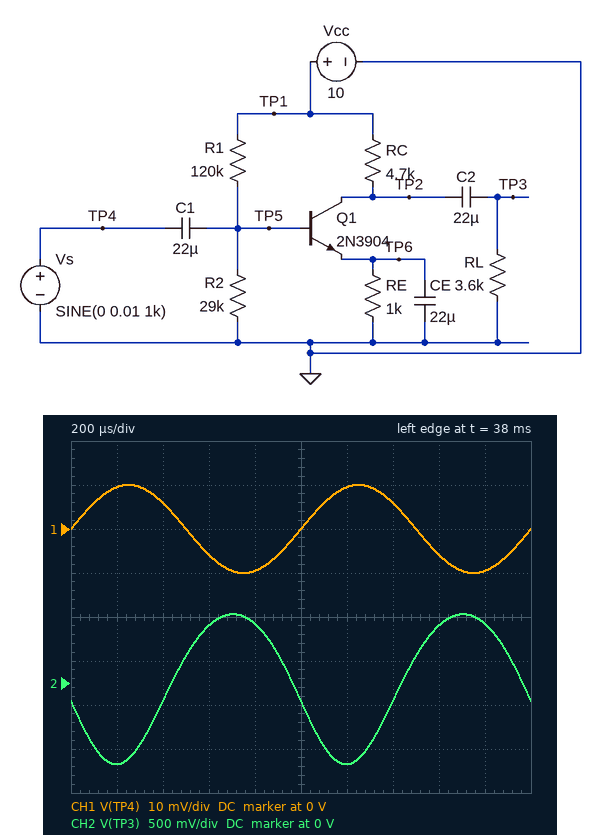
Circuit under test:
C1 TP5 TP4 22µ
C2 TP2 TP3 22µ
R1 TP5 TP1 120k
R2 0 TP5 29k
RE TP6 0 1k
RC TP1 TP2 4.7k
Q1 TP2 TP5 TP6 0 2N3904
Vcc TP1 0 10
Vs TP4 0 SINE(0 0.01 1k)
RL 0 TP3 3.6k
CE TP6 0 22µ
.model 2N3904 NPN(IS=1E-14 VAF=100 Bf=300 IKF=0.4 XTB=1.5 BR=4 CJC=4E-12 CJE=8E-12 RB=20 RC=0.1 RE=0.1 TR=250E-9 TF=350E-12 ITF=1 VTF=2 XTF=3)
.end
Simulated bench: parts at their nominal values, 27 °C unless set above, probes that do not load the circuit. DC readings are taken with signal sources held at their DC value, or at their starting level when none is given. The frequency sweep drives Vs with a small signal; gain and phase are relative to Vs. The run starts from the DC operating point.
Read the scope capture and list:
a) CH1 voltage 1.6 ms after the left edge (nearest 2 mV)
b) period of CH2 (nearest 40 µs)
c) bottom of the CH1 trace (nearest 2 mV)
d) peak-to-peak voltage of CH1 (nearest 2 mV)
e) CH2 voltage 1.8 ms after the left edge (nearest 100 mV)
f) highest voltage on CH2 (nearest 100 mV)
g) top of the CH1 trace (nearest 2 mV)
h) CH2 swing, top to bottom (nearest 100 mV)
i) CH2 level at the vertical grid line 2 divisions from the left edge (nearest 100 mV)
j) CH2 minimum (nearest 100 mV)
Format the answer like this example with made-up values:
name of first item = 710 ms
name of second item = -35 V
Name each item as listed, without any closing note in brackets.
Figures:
CH1 voltage 1.6 ms after the left edge = -6 mV
period of CH2 = 1.00 ms
bottom of the CH1 trace = -10 mV
peak-to-peak voltage of CH1 = 20 mV
CH2 voltage 1.8 ms after the left edge = 700 mV
highest voltage on CH2 = 800 mV
top of the CH1 trace = 10 mV
CH2 swing, top to bottom = 1.7 V
CH2 level at the vertical grid line 2 divisions from the left edge = -200 mV
CH2 minimum = -900 mV
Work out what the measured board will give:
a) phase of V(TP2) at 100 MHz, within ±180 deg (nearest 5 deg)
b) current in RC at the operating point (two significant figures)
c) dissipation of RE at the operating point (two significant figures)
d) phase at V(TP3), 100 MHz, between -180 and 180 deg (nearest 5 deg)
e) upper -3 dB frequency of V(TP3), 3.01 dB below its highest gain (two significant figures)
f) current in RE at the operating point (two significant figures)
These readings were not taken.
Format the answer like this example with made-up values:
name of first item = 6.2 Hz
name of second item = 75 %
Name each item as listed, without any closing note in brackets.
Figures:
phase of V(TP2) at 100 MHz, within ±180 deg = 85 deg
current in RC at the operating point = 1.2 mA
dissipation of RE at the operating point = 1.4 mW
phase at V(TP3), 100 MHz, between -180 and 180 deg = 85 deg
upper -3 dB frequency of V(TP3), 3.01 dB below its highest gain = 16 MHz
current in RE at the operating point = 1.2 mA
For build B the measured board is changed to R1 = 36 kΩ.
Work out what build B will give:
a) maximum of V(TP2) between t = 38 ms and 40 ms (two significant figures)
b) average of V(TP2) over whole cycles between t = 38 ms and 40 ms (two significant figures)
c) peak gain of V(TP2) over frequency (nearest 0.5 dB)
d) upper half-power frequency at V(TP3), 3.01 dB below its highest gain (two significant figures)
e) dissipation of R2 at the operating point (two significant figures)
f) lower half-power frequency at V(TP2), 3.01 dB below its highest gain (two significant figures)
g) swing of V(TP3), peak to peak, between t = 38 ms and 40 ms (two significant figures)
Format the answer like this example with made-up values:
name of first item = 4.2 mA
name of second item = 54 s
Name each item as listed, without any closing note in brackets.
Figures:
maximum of V(TP2) between t = 38 ms and 40 ms = 2.0 V
average of V(TP2) over whole cycles between t = 38 ms and 40 ms = 1.9 V
peak gain of V(TP2) over frequency = 7.0 dB
upper half-power frequency at V(TP3), 3.01 dB below its highest gain = 400 kHz
dissipation of R2 at the operating point = 220 µW
lower half-power frequency at V(TP2), 3.01 dB below its highest gain = 200 Hz
swing of V(TP3), peak to peak, between t = 38 ms and 40 ms = 120 mV
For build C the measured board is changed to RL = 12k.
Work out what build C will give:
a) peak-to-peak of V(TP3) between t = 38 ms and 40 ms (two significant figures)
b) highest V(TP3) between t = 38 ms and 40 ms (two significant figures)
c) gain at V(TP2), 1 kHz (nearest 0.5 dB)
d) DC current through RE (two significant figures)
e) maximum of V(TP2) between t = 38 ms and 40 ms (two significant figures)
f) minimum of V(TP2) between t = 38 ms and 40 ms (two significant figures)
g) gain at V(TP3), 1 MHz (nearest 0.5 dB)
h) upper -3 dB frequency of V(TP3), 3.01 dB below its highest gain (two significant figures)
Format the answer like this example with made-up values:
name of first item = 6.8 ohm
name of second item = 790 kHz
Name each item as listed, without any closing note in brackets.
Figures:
peak-to-peak of V(TP3) between t = 38 ms and 40 ms = 2.8 V
highest V(TP3) between t = 38 ms and 40 ms = 1.3 V
gain at V(TP2), 1 kHz = 43.0 dB
DC current through RE = 1.2 mA
maximum of V(TP2) between t = 38 ms and 40 ms = 5.7 V
minimum of V(TP2) between t = 38 ms and 40 ms = 2.9 V
gain at V(TP3), 1 MHz = 43.5 dB
upper -3 dB frequency of V(TP3), 3.01 dB below its highest gain = 10 MHz
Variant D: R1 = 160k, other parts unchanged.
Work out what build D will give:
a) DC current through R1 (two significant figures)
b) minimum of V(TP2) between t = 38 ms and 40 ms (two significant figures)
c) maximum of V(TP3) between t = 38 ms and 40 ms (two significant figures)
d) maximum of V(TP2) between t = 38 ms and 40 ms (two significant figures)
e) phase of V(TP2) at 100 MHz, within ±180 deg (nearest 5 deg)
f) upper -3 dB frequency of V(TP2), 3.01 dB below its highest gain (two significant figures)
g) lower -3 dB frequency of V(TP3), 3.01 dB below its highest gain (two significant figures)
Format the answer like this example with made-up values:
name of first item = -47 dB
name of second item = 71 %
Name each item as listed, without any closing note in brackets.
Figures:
DC current through R1 = 53 µA
minimum of V(TP2) between t = 38 ms and 40 ms = 5.5 V
maximum of V(TP3) between t = 38 ms and 40 ms = 550 mV
maximum of V(TP2) between t = 38 ms and 40 ms = 6.7 V
phase of V(TP2) at 100 MHz, within ±180 deg = 90 deg
upper -3 dB frequency of V(TP2), 3.01 dB below its highest gain = 23 MHz
lower -3 dB frequency of V(TP3), 3.01 dB below its highest gain = 230 Hz
